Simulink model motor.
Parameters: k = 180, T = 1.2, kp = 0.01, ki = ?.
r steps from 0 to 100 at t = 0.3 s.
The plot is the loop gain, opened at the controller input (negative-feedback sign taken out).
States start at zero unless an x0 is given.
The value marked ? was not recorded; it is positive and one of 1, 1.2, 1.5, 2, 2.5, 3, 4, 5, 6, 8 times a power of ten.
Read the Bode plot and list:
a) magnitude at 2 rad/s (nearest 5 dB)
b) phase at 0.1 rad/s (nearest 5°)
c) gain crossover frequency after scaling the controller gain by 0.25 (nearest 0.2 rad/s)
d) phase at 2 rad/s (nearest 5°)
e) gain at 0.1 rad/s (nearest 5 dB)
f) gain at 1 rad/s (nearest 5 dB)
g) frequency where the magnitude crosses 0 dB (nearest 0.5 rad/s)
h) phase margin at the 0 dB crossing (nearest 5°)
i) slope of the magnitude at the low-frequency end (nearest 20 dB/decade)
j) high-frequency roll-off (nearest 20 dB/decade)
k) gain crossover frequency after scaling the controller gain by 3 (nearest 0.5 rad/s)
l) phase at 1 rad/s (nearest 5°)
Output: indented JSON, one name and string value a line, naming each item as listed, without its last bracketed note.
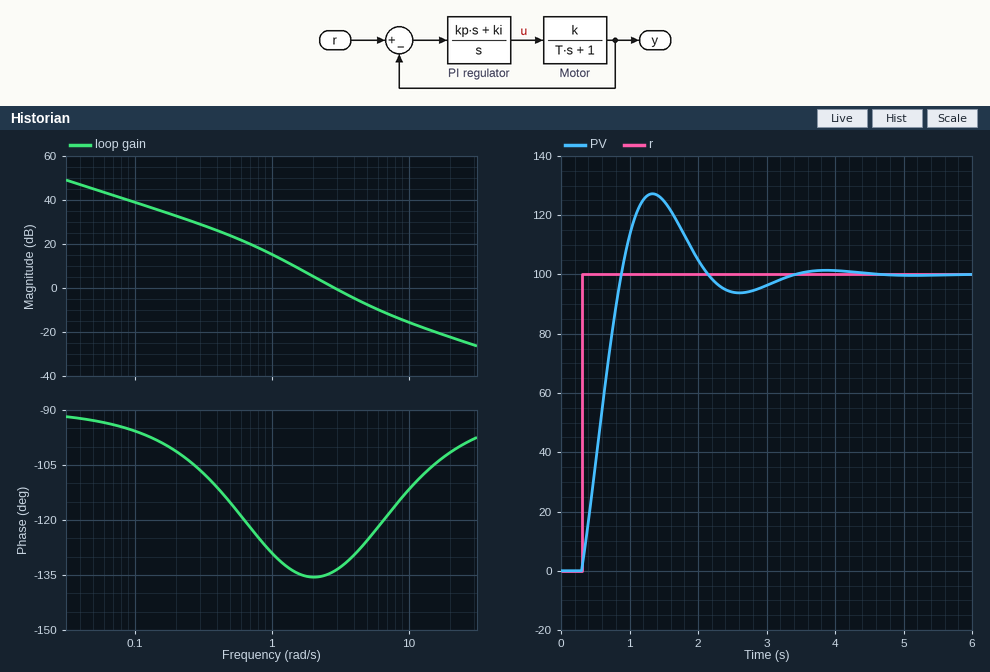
{
  "magnitude at 2 rad/s": "5 dB",
  "phase at 0.1 rad/s": "-95°",
  "gain crossover frequency after scaling the controller gain by 0.25": "1.2 rad/s",
  "phase at 2 rad/s": "-135°",
  "gain at 0.1 rad/s": "40 dB",
  "gain at 1 rad/s": "15 dB",
  "frequency where the magnitude crosses 0 dB": "3.0 rad/s",
  "phase margin at the 0 dB crossing": "45°",
  "slope of the magnitude at the low-frequency end": "-20 dB/decade",
  "high-frequency roll-off": "-20 dB/decade",
  "gain crossover frequency after scaling the controller gain by 3": "6.0 rad/s",
  "phase at 1 rad/s": "-130°"
}
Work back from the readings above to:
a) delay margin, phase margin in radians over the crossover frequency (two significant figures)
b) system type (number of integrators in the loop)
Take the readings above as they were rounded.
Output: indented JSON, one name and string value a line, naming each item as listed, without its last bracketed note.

{
  "delay margin, phase margin in radians over the crossover frequency": "0.26 s",
  "system type": "1"
}
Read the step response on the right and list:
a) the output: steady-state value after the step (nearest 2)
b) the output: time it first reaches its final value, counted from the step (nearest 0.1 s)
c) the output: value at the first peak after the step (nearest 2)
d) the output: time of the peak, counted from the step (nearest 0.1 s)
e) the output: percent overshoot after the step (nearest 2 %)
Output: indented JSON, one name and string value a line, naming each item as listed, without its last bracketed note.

{
  "the output: steady-state value after the step": "100",
  "the output: time it first reaches its final value, counted from the step": "0.6 s",
  "the output: value at the first peak after the step": "128",
  "the output: time of the peak, counted from the step": "1.0 s",
  "the output: percent overshoot after the step": "28 %"
}
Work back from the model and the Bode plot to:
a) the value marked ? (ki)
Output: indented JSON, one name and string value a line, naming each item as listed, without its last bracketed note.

{
  "the value marked ?": "0.05"
}
